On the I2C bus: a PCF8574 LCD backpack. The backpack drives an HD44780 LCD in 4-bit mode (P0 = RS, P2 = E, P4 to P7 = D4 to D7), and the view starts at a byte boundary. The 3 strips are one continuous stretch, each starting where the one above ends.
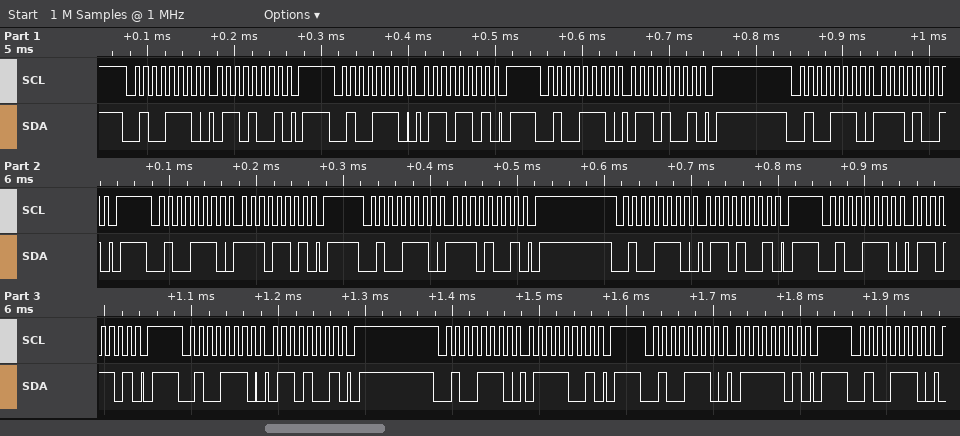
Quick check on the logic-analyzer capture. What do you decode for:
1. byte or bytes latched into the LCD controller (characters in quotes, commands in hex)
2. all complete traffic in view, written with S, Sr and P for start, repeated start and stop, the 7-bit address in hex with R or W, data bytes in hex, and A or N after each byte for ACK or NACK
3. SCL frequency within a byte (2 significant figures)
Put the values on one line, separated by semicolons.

'n'; S 27W A 69 A P S 27W A 6D A P S 27W A 69 A P S 27W A E9 A P S 27W A ED A P S 27W A E9 A P S 27W A 69 A P S 27W A 6D A P S 27W A 69 A P S 27W A 79 A P S 27W A 7D A P S 27W A; 100 kHz
